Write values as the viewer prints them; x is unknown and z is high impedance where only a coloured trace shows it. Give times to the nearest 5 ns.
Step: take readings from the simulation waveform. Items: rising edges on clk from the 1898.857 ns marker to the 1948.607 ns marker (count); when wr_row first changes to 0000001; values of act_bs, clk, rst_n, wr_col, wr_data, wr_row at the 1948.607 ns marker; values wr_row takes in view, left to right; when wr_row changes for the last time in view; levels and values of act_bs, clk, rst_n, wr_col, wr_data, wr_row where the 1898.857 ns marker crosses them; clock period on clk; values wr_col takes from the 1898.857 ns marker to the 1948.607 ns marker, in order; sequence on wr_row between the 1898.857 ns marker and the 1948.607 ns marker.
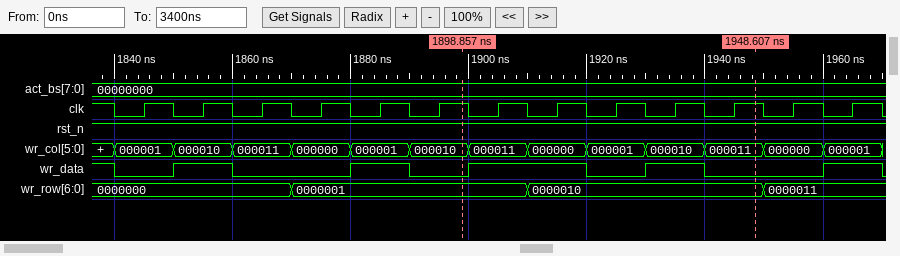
5
1870 ns
act_bs=00000000, clk=1, rst_n=1, wr_col=000011, wr_data=0, wr_row=0000010
0000000, 0000001, 0000010, 0000011
1950 ns
act_bs=00000000, clk=1, rst_n=1, wr_col=000010, wr_data=0, wr_row=0000001
10 ns
000010, 000011, 000000, 000001, 000010, 000011
0000001, 0000010
